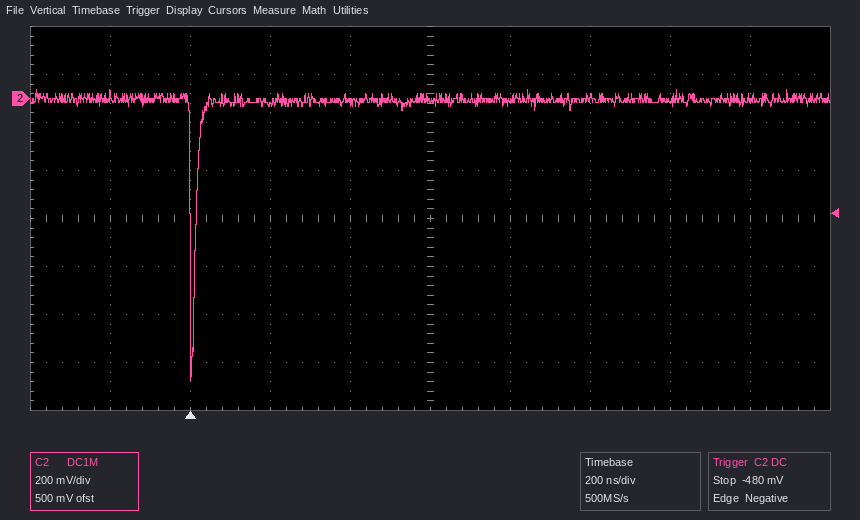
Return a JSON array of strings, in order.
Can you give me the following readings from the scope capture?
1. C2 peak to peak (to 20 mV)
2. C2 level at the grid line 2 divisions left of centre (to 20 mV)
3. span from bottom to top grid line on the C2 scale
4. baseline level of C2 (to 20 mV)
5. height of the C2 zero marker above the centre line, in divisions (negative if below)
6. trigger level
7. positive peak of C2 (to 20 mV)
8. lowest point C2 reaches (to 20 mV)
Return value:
["1.22 V", "-20 mV", "1.6 V", "0 mV", "+2.5 div", "-480 mV", "40 mV", "-1.18 V"]
